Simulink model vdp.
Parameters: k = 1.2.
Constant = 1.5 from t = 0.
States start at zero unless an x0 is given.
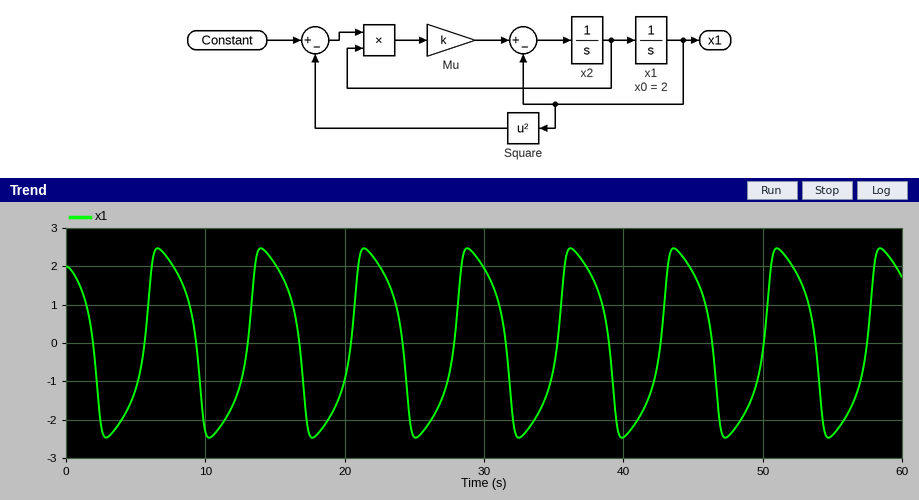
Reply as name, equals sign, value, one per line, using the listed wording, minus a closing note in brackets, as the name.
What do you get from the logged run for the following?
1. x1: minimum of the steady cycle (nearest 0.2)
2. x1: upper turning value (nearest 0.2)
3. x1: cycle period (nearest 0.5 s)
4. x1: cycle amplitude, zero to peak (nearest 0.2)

x1: minimum of the steady cycle = -2.4
x1: upper turning value = 2.4
x1: cycle period = 7.5 s
x1: cycle amplitude, zero to peak = 2.4
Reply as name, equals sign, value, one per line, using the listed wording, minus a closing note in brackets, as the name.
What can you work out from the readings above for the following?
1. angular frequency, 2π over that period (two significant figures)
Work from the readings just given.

angular frequency, 2π over that period = 0.84 rad/s
